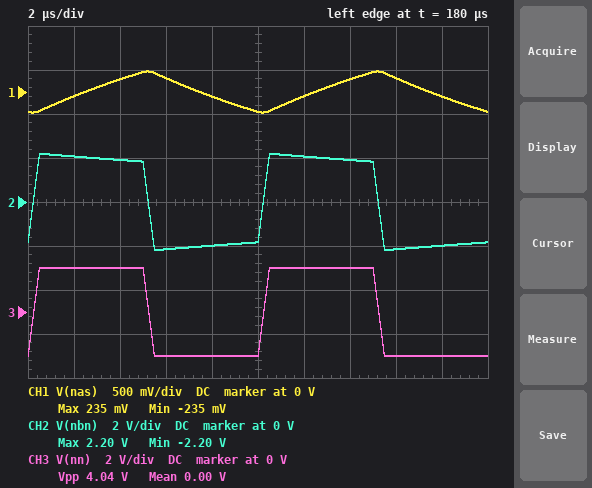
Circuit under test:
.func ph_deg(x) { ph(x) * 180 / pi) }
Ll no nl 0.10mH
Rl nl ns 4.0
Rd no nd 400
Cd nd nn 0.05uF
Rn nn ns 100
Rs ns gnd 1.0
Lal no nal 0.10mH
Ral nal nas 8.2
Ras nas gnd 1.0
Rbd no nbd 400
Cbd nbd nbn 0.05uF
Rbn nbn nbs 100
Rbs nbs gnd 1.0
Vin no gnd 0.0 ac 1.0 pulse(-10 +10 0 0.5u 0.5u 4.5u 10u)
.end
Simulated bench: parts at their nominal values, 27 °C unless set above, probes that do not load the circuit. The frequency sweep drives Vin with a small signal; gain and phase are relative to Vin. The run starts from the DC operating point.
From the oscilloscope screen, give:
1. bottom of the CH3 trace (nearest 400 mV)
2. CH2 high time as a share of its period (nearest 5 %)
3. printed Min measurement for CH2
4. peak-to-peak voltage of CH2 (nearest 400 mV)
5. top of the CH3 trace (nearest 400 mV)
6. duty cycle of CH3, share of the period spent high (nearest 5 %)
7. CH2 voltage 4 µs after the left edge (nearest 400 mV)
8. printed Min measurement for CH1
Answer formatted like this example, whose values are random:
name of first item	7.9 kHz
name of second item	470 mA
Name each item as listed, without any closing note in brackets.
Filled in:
bottom of the CH3 trace	-2.0 V
CH2 high time as a share of its period	50 %
printed Min measurement for CH2	-2.20 V
peak-to-peak voltage of CH2	4.4 V
top of the CH3 trace	2.0 V
duty cycle of CH3, share of the period spent high	50 %
CH2 voltage 4 µs after the left edge	2.0 V
printed Min measurement for CH1	-235 mV
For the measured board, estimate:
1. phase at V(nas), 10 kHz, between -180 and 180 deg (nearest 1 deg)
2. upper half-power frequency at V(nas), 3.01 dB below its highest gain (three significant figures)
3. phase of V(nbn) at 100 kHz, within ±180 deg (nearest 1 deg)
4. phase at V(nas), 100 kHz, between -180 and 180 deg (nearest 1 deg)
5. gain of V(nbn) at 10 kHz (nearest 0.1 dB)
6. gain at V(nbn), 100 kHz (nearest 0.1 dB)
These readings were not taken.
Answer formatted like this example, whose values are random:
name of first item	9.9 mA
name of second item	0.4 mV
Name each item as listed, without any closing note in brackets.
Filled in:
phase at V(nas), 10 kHz, between -180 and 180 deg	-34 deg
upper half-power frequency at V(nas), 3.01 dB below its highest gain	14.6 kHz
phase of V(nbn) at 100 kHz, within ±180 deg	4 deg
phase at V(nas), 100 kHz, between -180 and 180 deg	-82 deg
gain of V(nbn) at 10 kHz	-15.4 dB
gain at V(nbn), 100 kHz	-13.9 dB
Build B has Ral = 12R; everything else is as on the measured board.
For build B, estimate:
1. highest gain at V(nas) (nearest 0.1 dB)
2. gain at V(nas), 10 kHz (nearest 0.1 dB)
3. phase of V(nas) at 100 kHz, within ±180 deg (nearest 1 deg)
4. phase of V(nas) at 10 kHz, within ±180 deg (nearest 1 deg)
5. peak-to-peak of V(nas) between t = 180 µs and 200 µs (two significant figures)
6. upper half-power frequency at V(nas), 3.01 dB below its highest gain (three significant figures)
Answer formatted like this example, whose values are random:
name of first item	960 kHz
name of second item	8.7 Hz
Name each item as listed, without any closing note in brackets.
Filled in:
highest gain at V(nas)	-22.3 dB
gain at V(nas), 10 kHz	-23.2 dB
phase of V(nas) at 100 kHz, within ±180 deg	-78 deg
phase of V(nas) at 10 kHz, within ±180 deg	-26 deg
peak-to-peak of V(nas) between t = 180 µs and 200 µs	460 mV
upper half-power frequency at V(nas), 3.01 dB below its highest gain	20.7 kHz
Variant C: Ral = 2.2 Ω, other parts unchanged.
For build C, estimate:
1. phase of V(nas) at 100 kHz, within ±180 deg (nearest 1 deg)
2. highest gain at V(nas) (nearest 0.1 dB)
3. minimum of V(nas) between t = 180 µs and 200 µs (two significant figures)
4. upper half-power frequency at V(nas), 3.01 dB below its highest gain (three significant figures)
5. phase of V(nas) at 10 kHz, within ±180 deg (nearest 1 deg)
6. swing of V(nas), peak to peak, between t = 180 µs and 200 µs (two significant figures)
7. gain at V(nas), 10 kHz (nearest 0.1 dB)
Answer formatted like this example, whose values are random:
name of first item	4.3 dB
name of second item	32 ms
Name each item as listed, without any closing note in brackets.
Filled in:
phase of V(nas) at 100 kHz, within ±180 deg	-87 deg
highest gain at V(nas)	-10.1 dB
minimum of V(nas) between t = 180 µs and 200 µs	-250 mV
upper half-power frequency at V(nas), 3.01 dB below its highest gain	5.09 kHz
phase of V(nas) at 10 kHz, within ±180 deg	-63 deg
swing of V(nas), peak to peak, between t = 180 µs and 200 µs	480 mV
gain at V(nas), 10 kHz	-17.0 dB
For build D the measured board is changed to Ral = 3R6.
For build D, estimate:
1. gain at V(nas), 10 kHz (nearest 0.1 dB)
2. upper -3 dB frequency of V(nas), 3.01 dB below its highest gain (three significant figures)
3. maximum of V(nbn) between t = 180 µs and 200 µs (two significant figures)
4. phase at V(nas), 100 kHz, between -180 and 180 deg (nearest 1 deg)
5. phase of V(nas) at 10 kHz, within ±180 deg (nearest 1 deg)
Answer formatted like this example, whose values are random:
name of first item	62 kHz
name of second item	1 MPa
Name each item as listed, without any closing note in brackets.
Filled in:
gain at V(nas), 10 kHz	-17.8 dB
upper -3 dB frequency of V(nas), 3.01 dB below its highest gain	7.32 kHz
maximum of V(nbn) between t = 180 µs and 200 µs	2.2 V
phase at V(nas), 100 kHz, between -180 and 180 deg	-86 deg
phase of V(nas) at 10 kHz, within ±180 deg	-54 deg
